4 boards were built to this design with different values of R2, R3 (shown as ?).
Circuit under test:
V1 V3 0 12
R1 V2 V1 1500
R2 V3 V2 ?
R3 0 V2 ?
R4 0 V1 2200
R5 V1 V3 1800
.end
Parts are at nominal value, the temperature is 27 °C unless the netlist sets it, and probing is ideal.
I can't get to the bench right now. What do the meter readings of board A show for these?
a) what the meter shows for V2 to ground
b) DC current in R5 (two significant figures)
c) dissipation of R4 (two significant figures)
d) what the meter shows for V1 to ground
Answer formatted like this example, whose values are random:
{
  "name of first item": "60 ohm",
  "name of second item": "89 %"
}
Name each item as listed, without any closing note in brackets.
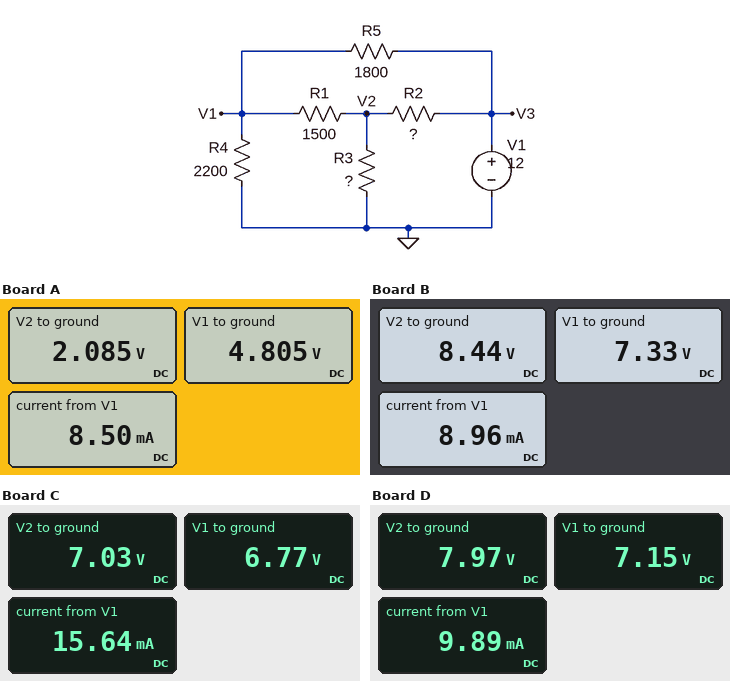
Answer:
{
  "what the meter shows for V2 to ground": "2.085 V",
  "DC current in R5": "4.0 mA",
  "dissipation of R4": "10 mW",
  "what the meter shows for V1 to ground": "4.805 V"
}
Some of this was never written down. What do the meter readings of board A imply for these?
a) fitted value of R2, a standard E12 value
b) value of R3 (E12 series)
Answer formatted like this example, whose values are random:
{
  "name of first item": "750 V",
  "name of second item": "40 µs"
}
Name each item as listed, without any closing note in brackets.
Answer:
{
  "fitted value of R2, a standard E12 value": "2.2 kΩ",
  "value of R3": "330 Ω"
}
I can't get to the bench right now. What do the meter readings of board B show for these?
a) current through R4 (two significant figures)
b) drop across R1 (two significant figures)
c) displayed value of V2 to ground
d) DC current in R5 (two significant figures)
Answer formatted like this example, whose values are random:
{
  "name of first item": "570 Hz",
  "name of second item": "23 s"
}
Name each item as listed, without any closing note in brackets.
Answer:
{
  "current through R4": "3.3 mA",
  "drop across R1": "1.1 V",
  "displayed value of V2 to ground": "8.44 V",
  "DC current in R5": "2.6 mA"
}
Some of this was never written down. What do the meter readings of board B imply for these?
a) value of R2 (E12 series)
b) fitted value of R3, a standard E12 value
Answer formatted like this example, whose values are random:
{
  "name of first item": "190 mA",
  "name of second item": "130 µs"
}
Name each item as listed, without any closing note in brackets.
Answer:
{
  "value of R2": "560 Ω",
  "fitted value of R3, a standard E12 value": "1.5 kΩ"
}
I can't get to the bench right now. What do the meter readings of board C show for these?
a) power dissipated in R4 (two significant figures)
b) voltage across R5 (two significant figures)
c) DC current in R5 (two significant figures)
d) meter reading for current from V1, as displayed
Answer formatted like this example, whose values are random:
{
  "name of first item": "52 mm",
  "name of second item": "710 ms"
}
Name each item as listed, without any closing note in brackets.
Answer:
{
  "power dissipated in R4": "21 mW",
  "voltage across R5": "5.2 V",
  "DC current in R5": "2.9 mA",
  "meter reading for current from V1, as displayed": "15.64 mA"
}
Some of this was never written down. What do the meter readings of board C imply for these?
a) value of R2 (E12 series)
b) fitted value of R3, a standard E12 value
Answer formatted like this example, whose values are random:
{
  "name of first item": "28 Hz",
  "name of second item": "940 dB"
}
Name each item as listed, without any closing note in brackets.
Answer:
{
  "value of R2": "390 Ω",
  "fitted value of R3, a standard E12 value": "560 Ω"
}
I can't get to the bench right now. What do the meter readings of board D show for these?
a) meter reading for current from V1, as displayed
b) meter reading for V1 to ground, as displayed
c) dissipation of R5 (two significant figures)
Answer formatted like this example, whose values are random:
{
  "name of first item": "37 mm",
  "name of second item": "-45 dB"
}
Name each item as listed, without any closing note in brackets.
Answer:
{
  "meter reading for current from V1, as displayed": "9.89 mA",
  "meter reading for V1 to ground, as displayed": "7.15 V",
  "dissipation of R5": "13 mW"
}
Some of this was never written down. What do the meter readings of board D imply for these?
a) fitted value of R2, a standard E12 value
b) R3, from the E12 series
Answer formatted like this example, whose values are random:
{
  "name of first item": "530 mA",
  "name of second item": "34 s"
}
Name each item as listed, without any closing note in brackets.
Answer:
{
  "fitted value of R2, a standard E12 value": "560 Ω",
  "R3, from the E12 series": "1.2 kΩ"
}
